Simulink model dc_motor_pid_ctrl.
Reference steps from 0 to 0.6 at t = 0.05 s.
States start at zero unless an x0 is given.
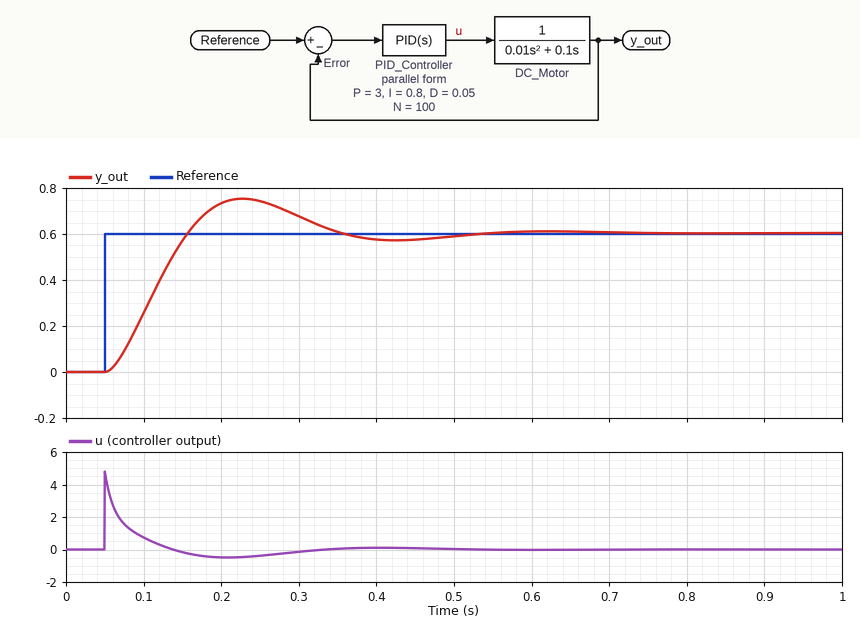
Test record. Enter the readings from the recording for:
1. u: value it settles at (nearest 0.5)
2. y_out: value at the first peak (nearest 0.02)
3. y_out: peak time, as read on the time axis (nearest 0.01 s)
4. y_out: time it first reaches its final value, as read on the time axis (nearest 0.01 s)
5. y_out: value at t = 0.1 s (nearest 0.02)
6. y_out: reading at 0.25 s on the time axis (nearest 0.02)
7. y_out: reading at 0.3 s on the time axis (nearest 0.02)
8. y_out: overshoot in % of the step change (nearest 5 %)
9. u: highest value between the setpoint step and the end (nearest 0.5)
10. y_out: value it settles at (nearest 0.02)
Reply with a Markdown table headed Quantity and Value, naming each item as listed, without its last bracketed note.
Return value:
| Quantity | Value |
|---|---|
| u: value it settles at | 0.0 |
| y_out: value at the first peak | 0.76 |
| y_out: peak time, as read on the time axis | 0.23 s |
| y_out: time it first reaches its final value, as read on the time axis | 0.16 s |
| y_out: value at t = 0.1 s | 0.26 |
| y_out: reading at 0.25 s on the time axis | 0.74 |
| y_out: reading at 0.3 s on the time axis | 0.68 |
| y_out: overshoot in % of the step change | 25 % |
| u: highest value between the setpoint step and the end | 5.0 |
| y_out: value it settles at | 0.60 |
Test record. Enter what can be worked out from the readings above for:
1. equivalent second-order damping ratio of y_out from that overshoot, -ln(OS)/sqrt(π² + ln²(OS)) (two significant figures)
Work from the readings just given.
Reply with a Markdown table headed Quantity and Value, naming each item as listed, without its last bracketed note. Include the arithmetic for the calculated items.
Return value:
| Quantity | Value |
|---|---|
| equivalent second-order damping ratio of y_out from that overshoot, -ln(OS)/sqrt(π² + ln²(OS)) | ln(0.25) = -1.386; 1.386 / sqrt(9.870 + 1.922) = 0.40 |
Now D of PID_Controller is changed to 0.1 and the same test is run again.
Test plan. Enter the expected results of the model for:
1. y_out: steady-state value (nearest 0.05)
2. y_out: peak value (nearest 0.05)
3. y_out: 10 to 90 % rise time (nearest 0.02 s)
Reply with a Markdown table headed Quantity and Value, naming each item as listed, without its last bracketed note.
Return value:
| Quantity | Value |
|---|---|
| y_out: steady-state value | 0.60 |
| y_out: peak value | 0.70 |
| y_out: 10 to 90 % rise time | 0.08 s |
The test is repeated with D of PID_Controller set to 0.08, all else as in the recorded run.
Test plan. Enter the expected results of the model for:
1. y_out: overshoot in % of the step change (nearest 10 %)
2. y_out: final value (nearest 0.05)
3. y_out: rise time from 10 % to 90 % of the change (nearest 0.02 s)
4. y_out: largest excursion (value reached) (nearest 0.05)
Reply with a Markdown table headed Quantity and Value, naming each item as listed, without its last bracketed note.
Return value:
| Quantity | Value |
|---|---|
| y_out: overshoot in % of the step change | 20 % |
| y_out: final value | 0.60 |
| y_out: rise time from 10 % to 90 % of the change | 0.08 s |
| y_out: largest excursion (value reached) | 0.70 |
